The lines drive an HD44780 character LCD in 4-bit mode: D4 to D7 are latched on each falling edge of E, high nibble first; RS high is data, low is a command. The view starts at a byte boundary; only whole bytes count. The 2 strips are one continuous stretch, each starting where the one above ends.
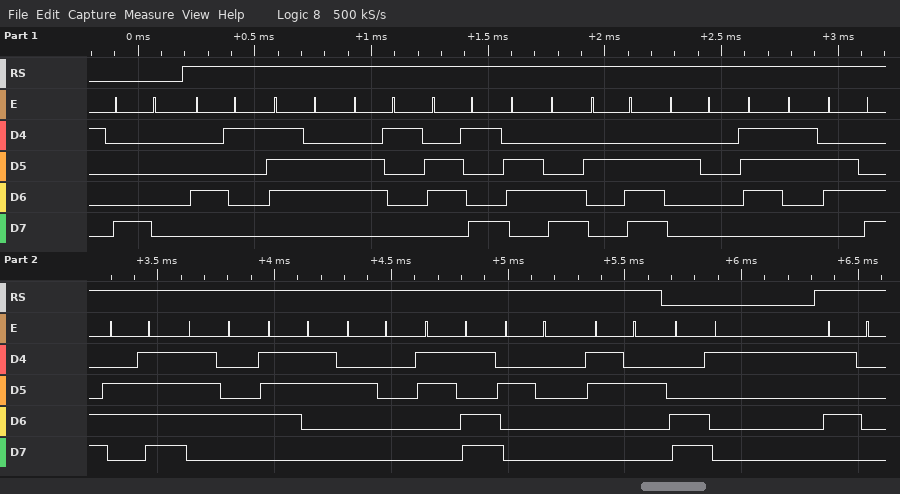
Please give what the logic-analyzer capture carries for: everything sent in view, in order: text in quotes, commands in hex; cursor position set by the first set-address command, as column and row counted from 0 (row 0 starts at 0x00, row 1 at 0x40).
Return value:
0x80 "Avail. slots = 2" 0xC1 "P"
column 0, row 0
